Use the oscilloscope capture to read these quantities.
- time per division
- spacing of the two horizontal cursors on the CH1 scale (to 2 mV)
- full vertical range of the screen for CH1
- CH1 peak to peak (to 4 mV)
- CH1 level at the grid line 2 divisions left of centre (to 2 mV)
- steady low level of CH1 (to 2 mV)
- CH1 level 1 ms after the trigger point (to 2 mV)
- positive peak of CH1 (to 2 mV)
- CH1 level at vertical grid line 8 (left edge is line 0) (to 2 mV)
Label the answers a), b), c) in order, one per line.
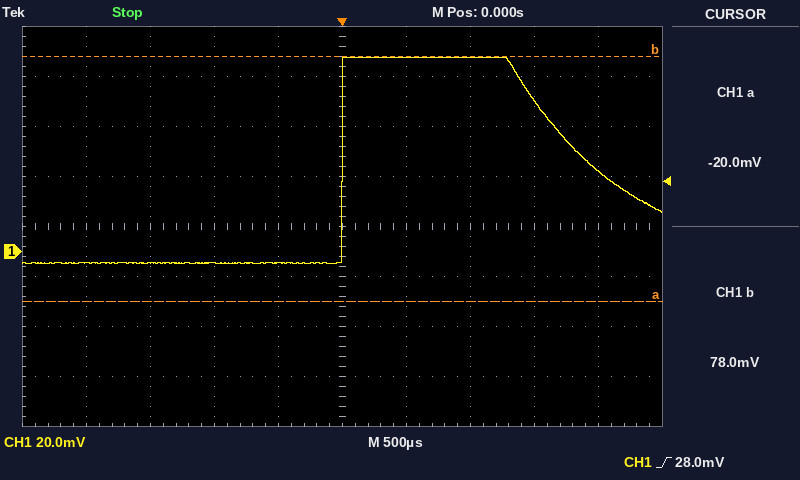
a) 500 µs
b) 98 mV
c) 160 mV
d) 84 mV
e) -4 mV
f) -4 mV
g) 78 mV
h) 78 mV
i) 60 mV
